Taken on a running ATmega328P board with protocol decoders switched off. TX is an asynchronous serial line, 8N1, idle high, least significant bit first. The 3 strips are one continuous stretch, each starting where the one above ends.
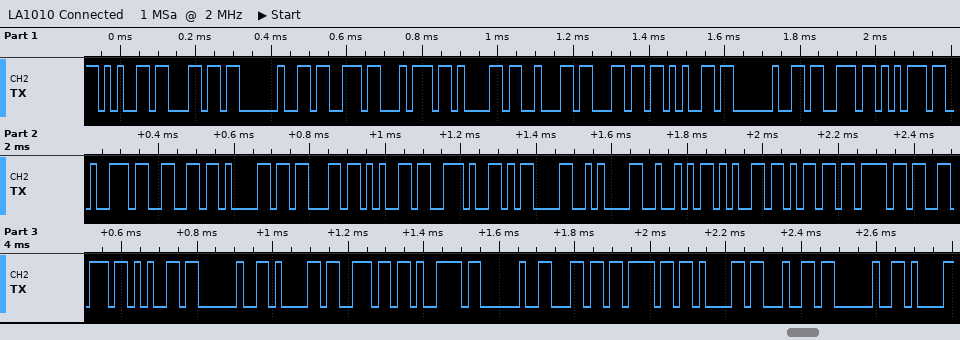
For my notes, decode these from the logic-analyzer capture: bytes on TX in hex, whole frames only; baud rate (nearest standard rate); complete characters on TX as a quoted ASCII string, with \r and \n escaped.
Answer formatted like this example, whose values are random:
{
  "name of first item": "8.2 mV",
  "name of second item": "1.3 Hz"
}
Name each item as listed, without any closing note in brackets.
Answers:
{
  "bytes on TX in hex, whole frames only": "65 6C 20 73 74 61 62 6C 65 20 73 75 72 66 61 63 65 2E 0D 0A 52 65 6D 6F 76 65 20 61 6E 79 20 6C 6F 61 64 20",
  "baud rate": "57600 baud",
  "complete characters on TX as a quoted ASCII string, with \\r and \\n escaped": "\"el stable surface.\\r\\nRemove any load \""
}
